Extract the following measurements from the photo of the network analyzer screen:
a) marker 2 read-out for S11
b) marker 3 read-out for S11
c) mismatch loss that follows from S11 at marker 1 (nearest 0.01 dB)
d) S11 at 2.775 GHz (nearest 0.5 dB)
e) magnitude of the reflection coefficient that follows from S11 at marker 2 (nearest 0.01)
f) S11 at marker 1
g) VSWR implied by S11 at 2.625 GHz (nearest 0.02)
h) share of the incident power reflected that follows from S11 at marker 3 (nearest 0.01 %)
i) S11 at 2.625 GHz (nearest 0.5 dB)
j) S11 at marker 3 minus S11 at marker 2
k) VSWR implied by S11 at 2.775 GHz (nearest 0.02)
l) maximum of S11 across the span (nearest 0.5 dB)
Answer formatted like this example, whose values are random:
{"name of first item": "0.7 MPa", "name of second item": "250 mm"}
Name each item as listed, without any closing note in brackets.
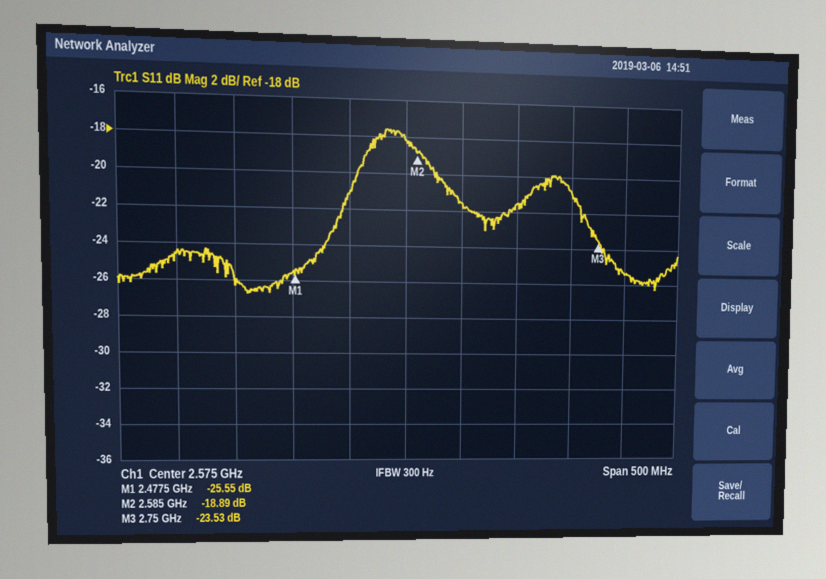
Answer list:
{"marker 2 read-out for S11": "-18.89 dB", "marker 3 read-out for S11": "-23.53 dB", "mismatch loss that follows from S11 at marker 1": "0.01 dB", "S11 at 2.775 GHz": "-25.5 dB", "magnitude of the reflection coefficient that follows from S11 at marker 2": "0.11", "S11 at marker 1": "-25.55 dB", "VSWR implied by S11 at 2.625 GHz": "1.18", "share of the incident power reflected that follows from S11 at marker 3": "0.44 %", "S11 at 2.625 GHz": "-21.5 dB", "S11 at marker 3 minus S11 at marker 2": "-4.64 dB", "VSWR implied by S11 at 2.775 GHz": "1.12", "maximum of S11 across the span": "-17.5 dB"}
